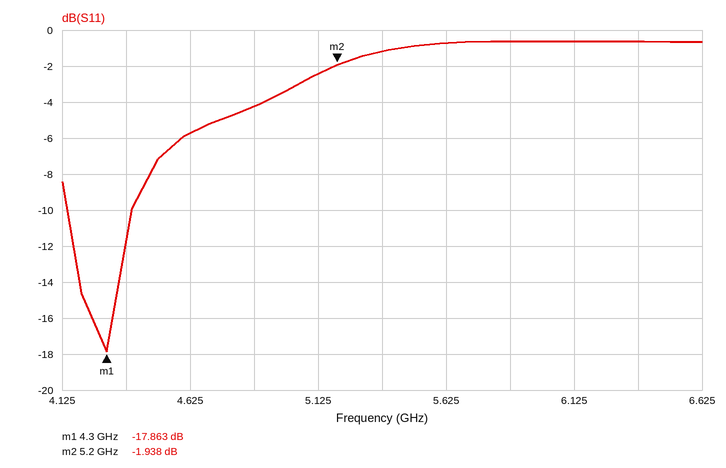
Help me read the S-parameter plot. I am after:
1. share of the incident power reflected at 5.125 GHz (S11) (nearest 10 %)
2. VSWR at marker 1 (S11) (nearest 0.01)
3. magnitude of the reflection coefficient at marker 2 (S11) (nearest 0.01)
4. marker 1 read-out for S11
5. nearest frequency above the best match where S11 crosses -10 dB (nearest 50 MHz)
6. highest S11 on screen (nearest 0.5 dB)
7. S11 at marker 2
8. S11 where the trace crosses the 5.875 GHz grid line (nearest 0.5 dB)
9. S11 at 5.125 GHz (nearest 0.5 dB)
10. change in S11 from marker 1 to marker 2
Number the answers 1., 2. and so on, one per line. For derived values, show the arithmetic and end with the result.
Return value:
1. 10^(-2.5/10) ≈ 56.2 %, so 60 % to the nearest 10 %
2. (1 + 0.1279)/(1 − 0.1279) ≈ 1.29
3. 10^(-1.938/20) ≈ 0.80
4. -17.863 dB
5. 4.40 GHz
6. -0.5 dB
7. -1.938 dB
8. -0.5 dB
9. -2.5 dB
10. -1.938 − (-17.863) = 15.925 dB
